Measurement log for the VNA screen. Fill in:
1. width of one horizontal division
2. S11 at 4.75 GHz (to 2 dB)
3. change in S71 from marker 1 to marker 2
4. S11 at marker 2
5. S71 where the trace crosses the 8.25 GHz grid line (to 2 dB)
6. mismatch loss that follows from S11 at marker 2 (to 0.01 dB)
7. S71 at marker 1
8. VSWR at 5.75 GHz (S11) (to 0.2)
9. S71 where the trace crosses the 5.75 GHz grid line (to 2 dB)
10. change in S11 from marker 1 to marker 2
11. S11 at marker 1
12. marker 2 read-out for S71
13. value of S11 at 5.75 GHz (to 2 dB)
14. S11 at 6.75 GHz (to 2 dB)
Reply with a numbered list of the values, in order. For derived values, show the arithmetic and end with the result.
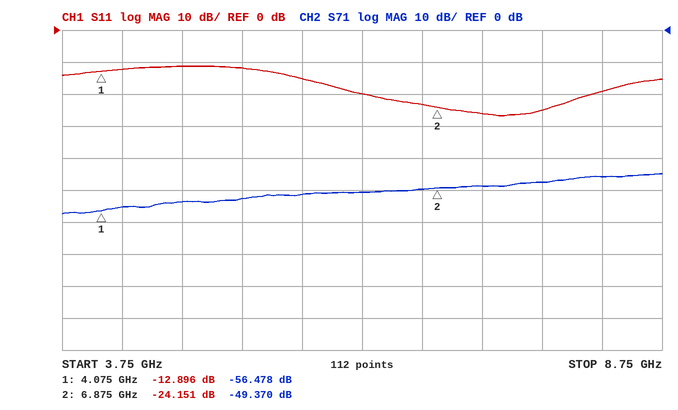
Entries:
1. 500 MHz
2. -12 dB
3. -49.37 − (-56.478) = 7.108 dB
4. -24.151 dB
5. -46 dB
6. −10 log10(1 − 10^(-24.151/10)) ≈ 0.02 dB
7. -56.478 dB
8. |Γ| = 10^(-16/20) = 0.1585; VSWR = (1 + 0.1585)/(1 − 0.1585) ≈ 1.4
9. -52 dB
10. -24.151 − (-12.896) = -11.255 dB
11. -12.896 dB
12. -49.370 dB
13. -16 dB
14. -24 dB
